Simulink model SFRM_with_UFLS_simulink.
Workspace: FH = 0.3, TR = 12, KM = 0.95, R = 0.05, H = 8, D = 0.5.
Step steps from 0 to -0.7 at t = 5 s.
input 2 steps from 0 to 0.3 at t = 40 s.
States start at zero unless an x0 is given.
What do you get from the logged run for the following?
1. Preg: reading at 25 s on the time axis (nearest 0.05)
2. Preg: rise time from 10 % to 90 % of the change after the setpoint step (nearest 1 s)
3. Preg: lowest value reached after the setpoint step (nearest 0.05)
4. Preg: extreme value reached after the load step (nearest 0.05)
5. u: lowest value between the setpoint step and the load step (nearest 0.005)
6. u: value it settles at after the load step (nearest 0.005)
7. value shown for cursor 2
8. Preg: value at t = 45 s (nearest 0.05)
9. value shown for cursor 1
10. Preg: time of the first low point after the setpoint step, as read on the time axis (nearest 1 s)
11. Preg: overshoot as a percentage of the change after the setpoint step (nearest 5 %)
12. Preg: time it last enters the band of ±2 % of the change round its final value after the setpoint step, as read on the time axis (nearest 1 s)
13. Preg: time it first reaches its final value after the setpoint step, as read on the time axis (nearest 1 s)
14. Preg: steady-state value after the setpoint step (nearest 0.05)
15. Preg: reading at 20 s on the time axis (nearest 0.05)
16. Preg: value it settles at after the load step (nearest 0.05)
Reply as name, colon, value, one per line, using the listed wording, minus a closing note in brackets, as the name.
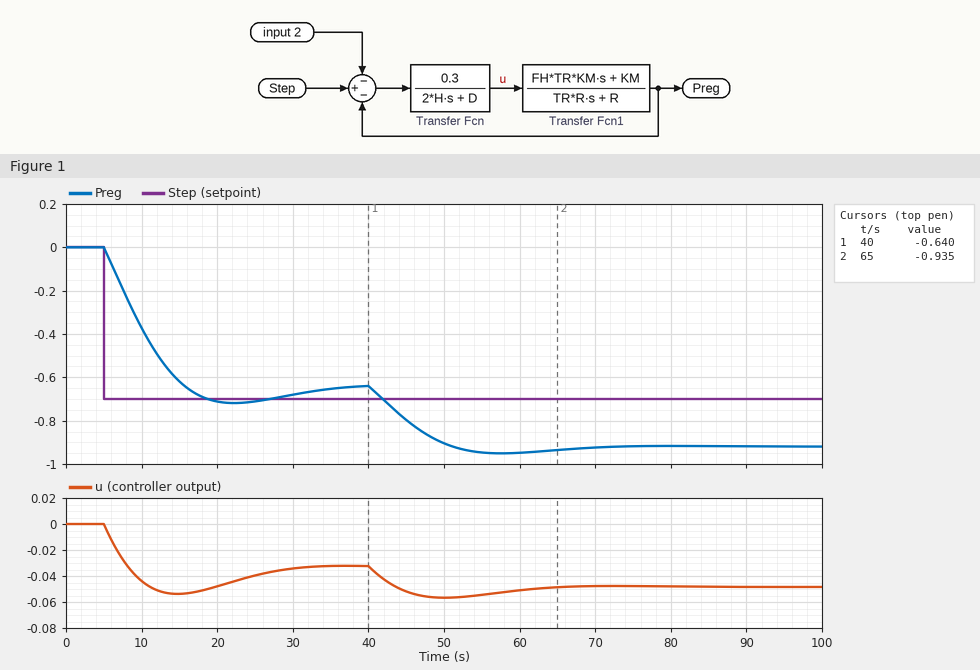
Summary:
Preg: reading at 25 s on the time axis: -0.70
Preg: rise time from 10 % to 90 % of the change after the setpoint step: 8 s
Preg: lowest value reached after the setpoint step: -0.70
Preg: extreme value reached after the load step: -0.95
u: lowest value between the setpoint step and the load step: -0.055
u: value it settles at after the load step: -0.050
value shown for cursor 2: -0.935
Preg: value at t = 45 s: -0.80
value shown for cursor 1: -0.640
Preg: time of the first low point after the setpoint step, as read on the time axis: 22 s
Preg: overshoot as a percentage of the change after the setpoint step: 10 %
Preg: time it last enters the band of ±2 % of the change round its final value after the setpoint step, as read on the time axis: 34 s
Preg: time it first reaches its final value after the setpoint step, as read on the time axis: 16 s
Preg: steady-state value after the setpoint step: -0.65
Preg: reading at 20 s on the time axis: -0.70
Preg: value it settles at after the load step: -0.90
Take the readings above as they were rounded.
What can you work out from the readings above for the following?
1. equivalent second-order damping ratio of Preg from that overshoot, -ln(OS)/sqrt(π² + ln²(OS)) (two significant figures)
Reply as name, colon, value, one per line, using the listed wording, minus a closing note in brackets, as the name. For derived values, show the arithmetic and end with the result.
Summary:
equivalent second-order damping ratio of Preg from that overshoot, -ln(OS)/sqrt(π² + ln²(OS)): ln(0.1) = -2.303; 2.303 / sqrt(9.870 + 5.302) = 0.59
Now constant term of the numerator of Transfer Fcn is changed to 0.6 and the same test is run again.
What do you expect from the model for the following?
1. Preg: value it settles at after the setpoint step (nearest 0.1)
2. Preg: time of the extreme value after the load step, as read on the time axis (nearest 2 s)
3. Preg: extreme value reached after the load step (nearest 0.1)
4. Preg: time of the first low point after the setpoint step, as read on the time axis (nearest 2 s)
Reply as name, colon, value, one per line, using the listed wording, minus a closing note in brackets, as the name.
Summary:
Preg: value it settles at after the setpoint step: -0.7
Preg: time of the extreme value after the load step, as read on the time axis: 52 s
Preg: extreme value reached after the load step: -1.0
Preg: time of the first low point after the setpoint step, as read on the time axis: 16 s
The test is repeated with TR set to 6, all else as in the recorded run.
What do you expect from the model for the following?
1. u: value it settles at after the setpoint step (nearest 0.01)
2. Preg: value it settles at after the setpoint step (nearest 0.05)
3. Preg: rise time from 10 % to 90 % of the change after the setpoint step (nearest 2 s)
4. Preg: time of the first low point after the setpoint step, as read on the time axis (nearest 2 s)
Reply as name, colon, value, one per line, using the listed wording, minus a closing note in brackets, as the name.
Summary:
u: value it settles at after the setpoint step: -0.03
Preg: value it settles at after the setpoint step: -0.65
Preg: rise time from 10 % to 90 % of the change after the setpoint step: 6 s
Preg: time of the first low point after the setpoint step, as read on the time axis: 18 s
